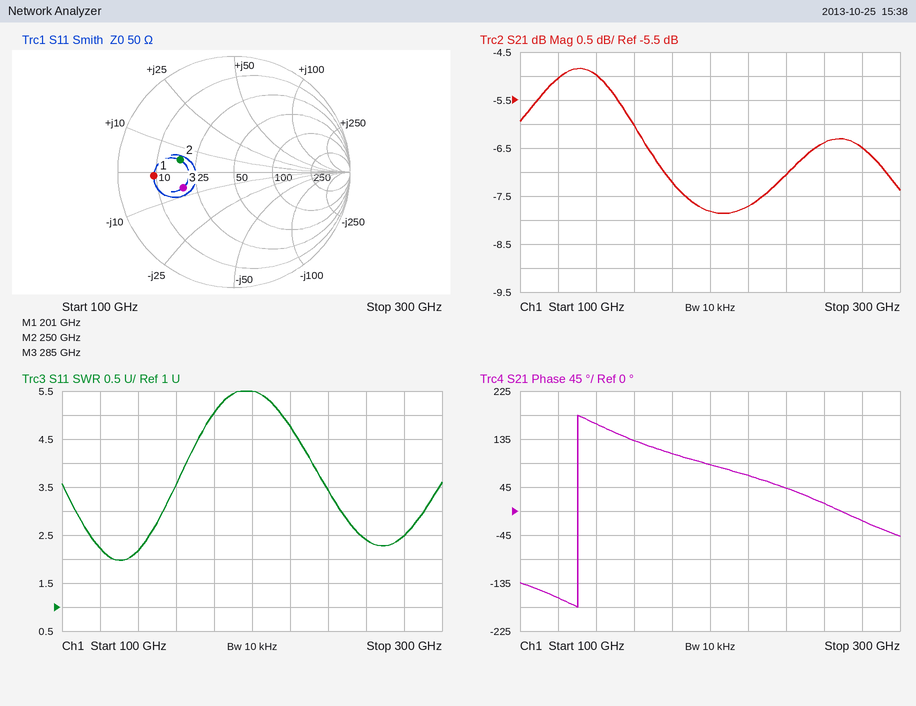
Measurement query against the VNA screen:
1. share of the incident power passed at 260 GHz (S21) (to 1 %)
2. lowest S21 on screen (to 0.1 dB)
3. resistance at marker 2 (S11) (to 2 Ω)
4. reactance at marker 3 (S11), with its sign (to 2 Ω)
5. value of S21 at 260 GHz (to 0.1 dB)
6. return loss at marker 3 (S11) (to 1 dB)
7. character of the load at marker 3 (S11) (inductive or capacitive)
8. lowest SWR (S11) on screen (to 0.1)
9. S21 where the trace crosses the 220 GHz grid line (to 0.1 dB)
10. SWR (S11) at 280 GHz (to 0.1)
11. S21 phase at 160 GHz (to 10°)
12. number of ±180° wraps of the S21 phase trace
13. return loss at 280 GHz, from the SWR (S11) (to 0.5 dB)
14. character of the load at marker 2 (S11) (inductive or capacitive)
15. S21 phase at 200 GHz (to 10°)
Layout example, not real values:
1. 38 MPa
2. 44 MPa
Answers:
1. 23 %
2. -7.9 dB
3. 18 Ω
4. -6 Ω
5. -6.4 dB
6. 7 dB
7. capacitive
8. 2.0
9. -7.7 dB
10. 2.5
11. 130°
12. 1
13. 7.5 dB
14. inductive
15. 90°
